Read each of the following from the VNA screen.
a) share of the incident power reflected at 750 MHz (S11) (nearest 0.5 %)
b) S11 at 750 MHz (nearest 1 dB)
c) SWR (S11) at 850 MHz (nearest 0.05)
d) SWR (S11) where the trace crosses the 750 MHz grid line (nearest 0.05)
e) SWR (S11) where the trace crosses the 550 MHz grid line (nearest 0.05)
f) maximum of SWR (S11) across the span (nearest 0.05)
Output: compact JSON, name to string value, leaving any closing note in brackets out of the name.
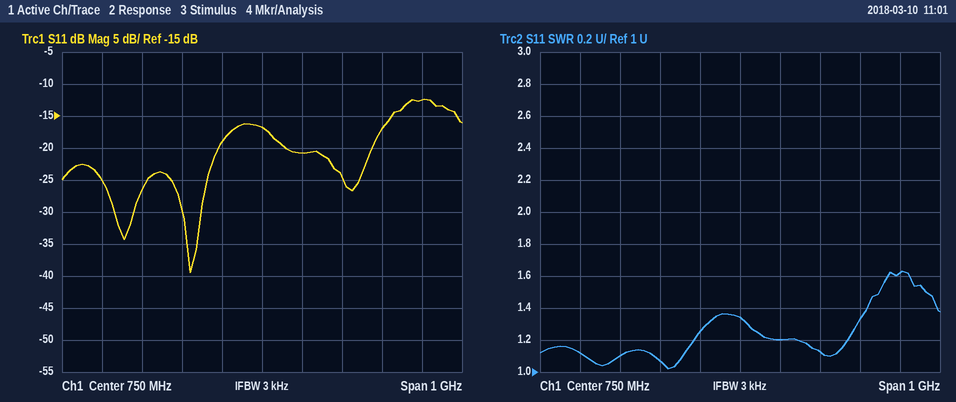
{"share of the incident power reflected at 750 MHz (S11)": "2.0 %", "S11 at 750 MHz": "-17 dB", "SWR (S11) at 850 MHz": "1.20", "SWR (S11) where the trace crosses the 750 MHz grid line": "1.35", "SWR (S11) where the trace crosses the 550 MHz grid line": "1.05", "maximum of SWR (S11) across the span": "1.65"}
